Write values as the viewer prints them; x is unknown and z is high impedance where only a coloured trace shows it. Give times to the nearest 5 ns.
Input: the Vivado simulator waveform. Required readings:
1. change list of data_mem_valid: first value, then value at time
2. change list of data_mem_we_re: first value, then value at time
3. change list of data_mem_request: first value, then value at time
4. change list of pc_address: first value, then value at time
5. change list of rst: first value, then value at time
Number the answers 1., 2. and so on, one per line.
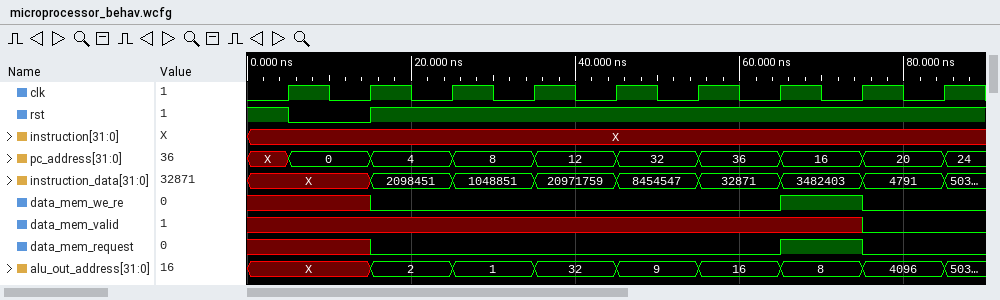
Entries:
1. x, 0 at 75 ns
2. x, 0 at 15 ns, 1 at 65 ns, 0 at 75 ns
3. x, 0 at 15 ns, 1 at 65 ns, 0 at 75 ns
4. X, 0 at 5 ns, 4 at 15 ns, 8 at 25 ns, 12 at 35 ns, 32 at 45 ns, 36 at 55 ns, 16 at 65 ns, 20 at 75 ns, 24 at 85 ns
5. 1, 0 at 5 ns, 1 at 15 ns
